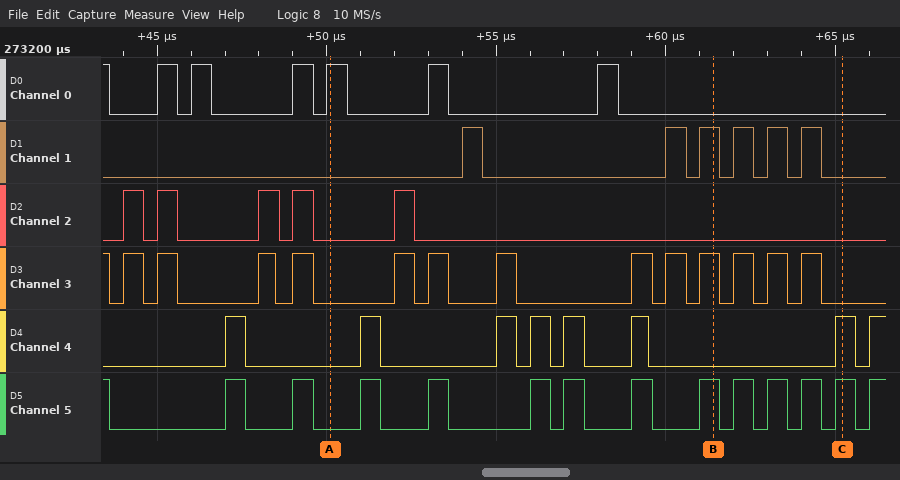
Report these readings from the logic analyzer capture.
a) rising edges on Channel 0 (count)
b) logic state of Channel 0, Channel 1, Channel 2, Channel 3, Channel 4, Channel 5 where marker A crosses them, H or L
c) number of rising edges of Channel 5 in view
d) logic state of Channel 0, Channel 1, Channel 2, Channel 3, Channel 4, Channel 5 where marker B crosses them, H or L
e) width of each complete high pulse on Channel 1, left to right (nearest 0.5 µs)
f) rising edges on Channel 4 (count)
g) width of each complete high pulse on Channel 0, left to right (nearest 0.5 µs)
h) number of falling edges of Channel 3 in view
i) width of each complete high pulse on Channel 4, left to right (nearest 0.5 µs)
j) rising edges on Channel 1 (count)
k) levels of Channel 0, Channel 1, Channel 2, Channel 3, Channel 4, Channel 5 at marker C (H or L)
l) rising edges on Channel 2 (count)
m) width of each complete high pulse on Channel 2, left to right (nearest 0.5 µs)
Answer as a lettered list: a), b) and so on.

a) 6
b) Channel 0=H, Channel 1=L, Channel 2=L, Channel 3=L, Channel 4=L, Channel 5=L
c) 13
d) Channel 0=L, Channel 1=H, Channel 2=L, Channel 3=H, Channel 4=L, Channel 5=H
e) 0.5 µs, 0.5 µs, 0.5 µs, 0.5 µs, 0.5 µs, 0.5 µs
f) 8
g) 0.5 µs, 0.5 µs, 0.5 µs, 0.5 µs, 0.5 µs, 0.5 µs
h) 14
i) 0.5 µs, 0.5 µs, 0.5 µs, 0.5 µs, 0.5 µs, 0.5 µs, 0.5 µs
j) 6
k) Channel 0=L, Channel 1=L, Channel 2=L, Channel 3=L, Channel 4=H, Channel 5=H
l) 5
m) 0.5 µs, 0.5 µs, 0.5 µs, 0.5 µs, 0.5 µs
